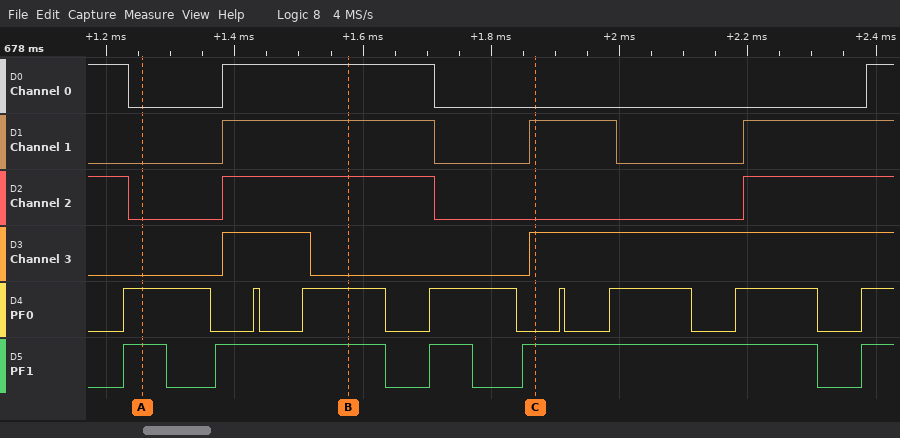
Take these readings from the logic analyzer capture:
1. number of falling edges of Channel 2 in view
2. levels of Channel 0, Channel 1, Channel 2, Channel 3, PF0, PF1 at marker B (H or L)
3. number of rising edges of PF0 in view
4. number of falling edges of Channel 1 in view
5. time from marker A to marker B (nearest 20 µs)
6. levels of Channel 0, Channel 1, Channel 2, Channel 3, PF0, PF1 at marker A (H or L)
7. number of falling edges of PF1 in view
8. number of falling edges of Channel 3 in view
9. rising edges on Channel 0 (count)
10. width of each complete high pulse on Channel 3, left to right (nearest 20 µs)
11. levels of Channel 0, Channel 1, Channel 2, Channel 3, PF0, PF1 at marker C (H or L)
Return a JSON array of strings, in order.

["2", "Channel 0=H, Channel 1=H, Channel 2=H, Channel 3=L, PF0=H, PF1=H", "8", "2", "320 µs", "Channel 0=L, Channel 1=L, Channel 2=L, Channel 3=L, PF0=H, PF1=H", "4", "1", "2", "140 µs", "Channel 0=L, Channel 1=H, Channel 2=L, Channel 3=H, PF0=L, PF1=H"]
